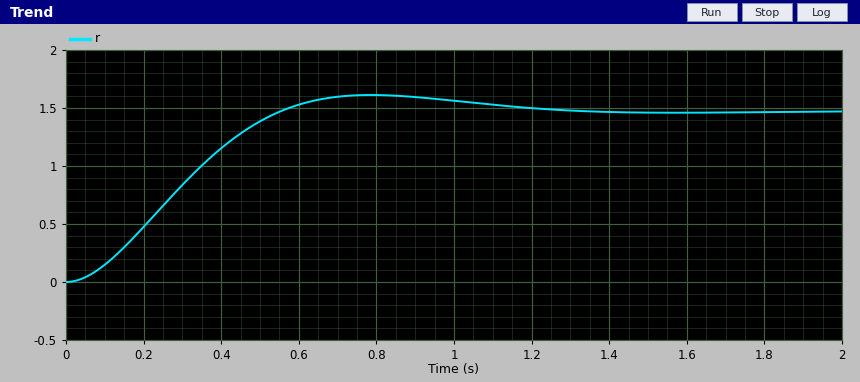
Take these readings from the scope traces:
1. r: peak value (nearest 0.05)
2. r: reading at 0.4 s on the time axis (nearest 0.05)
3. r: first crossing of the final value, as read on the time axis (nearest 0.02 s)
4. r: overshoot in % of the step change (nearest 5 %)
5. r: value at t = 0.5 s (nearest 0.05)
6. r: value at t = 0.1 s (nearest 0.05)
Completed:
1.60
1.15
0.56 s
10 %
1.40
0.15
